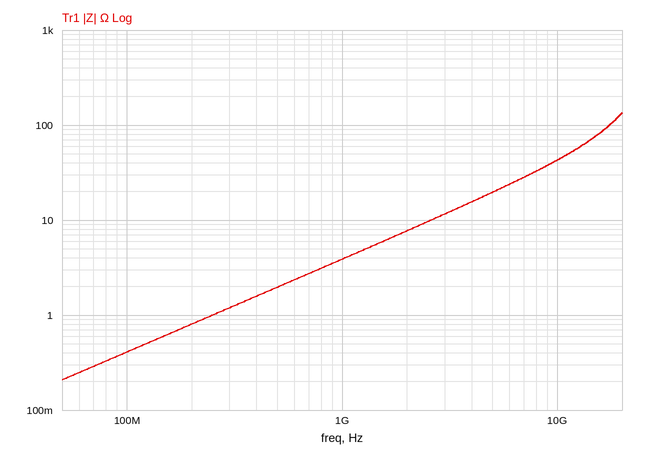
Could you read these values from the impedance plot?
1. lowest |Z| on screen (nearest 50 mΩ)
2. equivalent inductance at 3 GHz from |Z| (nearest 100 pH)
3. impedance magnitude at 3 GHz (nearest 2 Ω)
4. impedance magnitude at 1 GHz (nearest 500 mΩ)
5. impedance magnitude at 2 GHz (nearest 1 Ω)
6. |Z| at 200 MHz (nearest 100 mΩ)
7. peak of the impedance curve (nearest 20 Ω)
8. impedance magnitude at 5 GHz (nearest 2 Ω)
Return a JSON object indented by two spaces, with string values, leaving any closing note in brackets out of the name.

{
  "lowest |Z| on screen": "200 mΩ",
  "equivalent inductance at 3 GHz from |Z|": "600 pH",
  "impedance magnitude at 3 GHz": "12 Ω",
  "impedance magnitude at 1 GHz": "4.0 Ω",
  "impedance magnitude at 2 GHz": "8 Ω",
  "|Z| at 200 MHz": "800 mΩ",
  "peak of the impedance curve": "140 Ω",
  "impedance magnitude at 5 GHz": "20 Ω"
}
